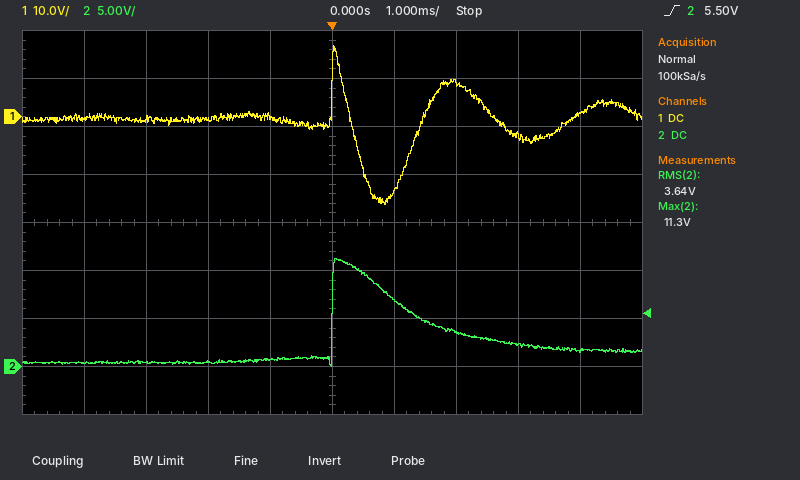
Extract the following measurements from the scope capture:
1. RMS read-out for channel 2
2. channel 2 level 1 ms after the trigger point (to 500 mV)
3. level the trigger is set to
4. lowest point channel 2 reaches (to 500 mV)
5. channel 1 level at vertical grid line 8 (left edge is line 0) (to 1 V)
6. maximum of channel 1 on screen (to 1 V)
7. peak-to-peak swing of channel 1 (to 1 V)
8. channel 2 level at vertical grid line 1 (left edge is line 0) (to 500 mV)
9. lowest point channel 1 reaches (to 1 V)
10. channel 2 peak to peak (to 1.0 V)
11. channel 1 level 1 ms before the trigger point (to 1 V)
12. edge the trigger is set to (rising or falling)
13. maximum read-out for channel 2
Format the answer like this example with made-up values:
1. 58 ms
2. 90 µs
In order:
1. 3.64 V
2. 7.0 V
3. 5.50 V
4. 0.0 V
5. -4 V
6. 15 V
7. 33 V
8. 500 mV
9. -18 V
10. 11.0 V
11. 0 V
12. rising
13. 11.3 V
